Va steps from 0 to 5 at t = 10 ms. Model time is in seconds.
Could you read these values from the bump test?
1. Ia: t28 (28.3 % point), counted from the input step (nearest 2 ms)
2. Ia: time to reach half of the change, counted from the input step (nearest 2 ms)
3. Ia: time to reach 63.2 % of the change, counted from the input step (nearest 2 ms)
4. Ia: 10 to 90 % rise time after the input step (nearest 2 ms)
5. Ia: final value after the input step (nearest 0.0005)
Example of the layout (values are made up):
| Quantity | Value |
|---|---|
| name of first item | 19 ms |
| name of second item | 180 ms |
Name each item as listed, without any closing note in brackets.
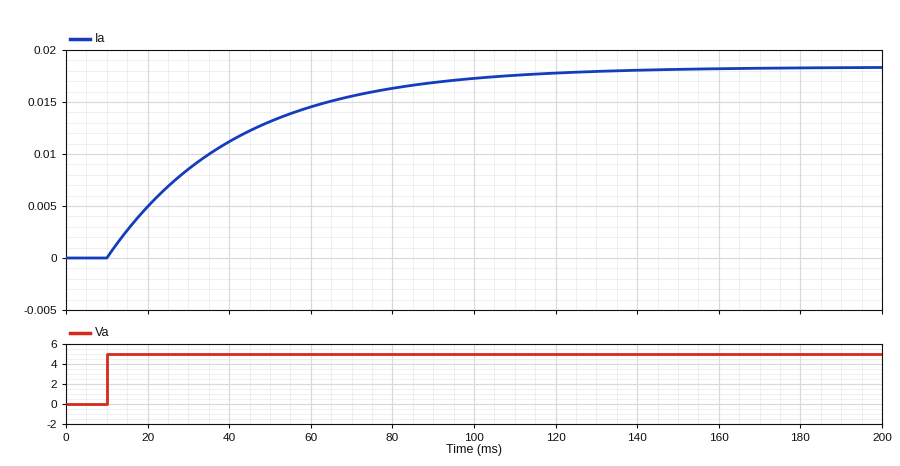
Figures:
| Quantity | Value |
|---|---|
| Ia: t28 (28.3 % point), counted from the input step | 10 ms |
| Ia: time to reach half of the change, counted from the input step | 22 ms |
| Ia: time to reach 63.2 % of the change, counted from the input step | 32 ms |
| Ia: 10 to 90 % rise time after the input step | 70 ms |
| Ia: final value after the input step | 0.0185 |
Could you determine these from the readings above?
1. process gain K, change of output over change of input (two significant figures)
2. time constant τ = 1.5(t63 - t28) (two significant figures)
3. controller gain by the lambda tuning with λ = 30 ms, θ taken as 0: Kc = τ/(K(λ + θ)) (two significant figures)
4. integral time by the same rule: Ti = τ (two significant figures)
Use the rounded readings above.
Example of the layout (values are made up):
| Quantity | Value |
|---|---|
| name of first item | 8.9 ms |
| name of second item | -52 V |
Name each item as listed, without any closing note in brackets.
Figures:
| Quantity | Value |
|---|---|
| process gain K, change of output over change of input | 0.0037 |
| time constant τ = 1.5(t63 - t28) | 33 ms |
| controller gain by the lambda tuning with λ = 30 ms, θ taken as 0: Kc = τ/(K(λ + θ)) | 300 |
| integral time by the same rule: Ti = τ | 33 ms |
